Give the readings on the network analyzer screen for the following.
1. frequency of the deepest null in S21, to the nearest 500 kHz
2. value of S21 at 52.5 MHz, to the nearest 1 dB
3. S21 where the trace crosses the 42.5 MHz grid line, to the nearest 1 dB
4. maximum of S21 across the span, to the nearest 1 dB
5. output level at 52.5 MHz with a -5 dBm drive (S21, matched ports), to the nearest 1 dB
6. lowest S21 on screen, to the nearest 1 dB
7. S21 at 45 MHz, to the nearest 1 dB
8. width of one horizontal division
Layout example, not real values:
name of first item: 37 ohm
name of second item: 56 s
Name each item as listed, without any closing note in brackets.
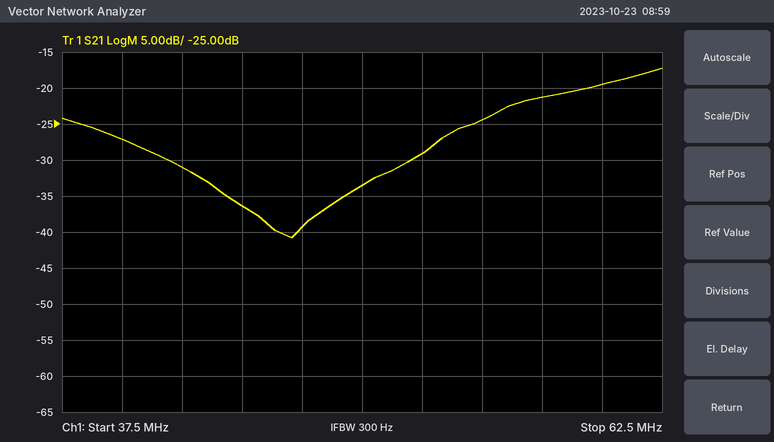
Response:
frequency of the deepest null in S21, to the nearest 500 kHz: 47.0 MHz
value of S21 at 52.5 MHz, to the nearest 1 dB: -29 dB
S21 where the trace crosses the 42.5 MHz grid line, to the nearest 1 dB: -31 dB
maximum of S21 across the span, to the nearest 1 dB: -17 dB
output level at 52.5 MHz with a -5 dBm drive (S21, matched ports), to the nearest 1 dB: -34 dBm
lowest S21 on screen, to the nearest 1 dB: -41 dB
S21 at 45 MHz, to the nearest 1 dB: -36 dB
width of one horizontal division: 2.5 MHz
